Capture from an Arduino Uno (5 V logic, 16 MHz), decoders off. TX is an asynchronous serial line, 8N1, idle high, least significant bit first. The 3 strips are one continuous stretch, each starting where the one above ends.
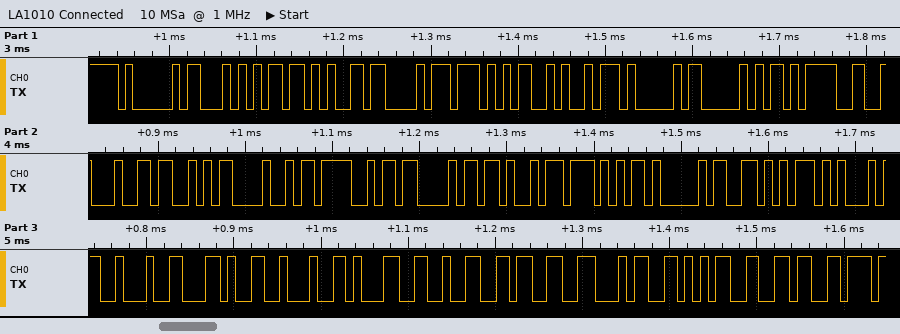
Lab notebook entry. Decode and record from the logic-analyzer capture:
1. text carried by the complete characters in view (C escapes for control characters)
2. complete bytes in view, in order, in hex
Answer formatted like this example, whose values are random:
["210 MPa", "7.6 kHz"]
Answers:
["\"AT+CWJAP=\\\"SHOCKWAVE\\\",\\\"123456\"", "41 54 2B 43 57 4A 41 50 3D 22 53 48 4F 43 4B 57 41 56 45 22 2C 22 31 32 33 34 35 36"]
